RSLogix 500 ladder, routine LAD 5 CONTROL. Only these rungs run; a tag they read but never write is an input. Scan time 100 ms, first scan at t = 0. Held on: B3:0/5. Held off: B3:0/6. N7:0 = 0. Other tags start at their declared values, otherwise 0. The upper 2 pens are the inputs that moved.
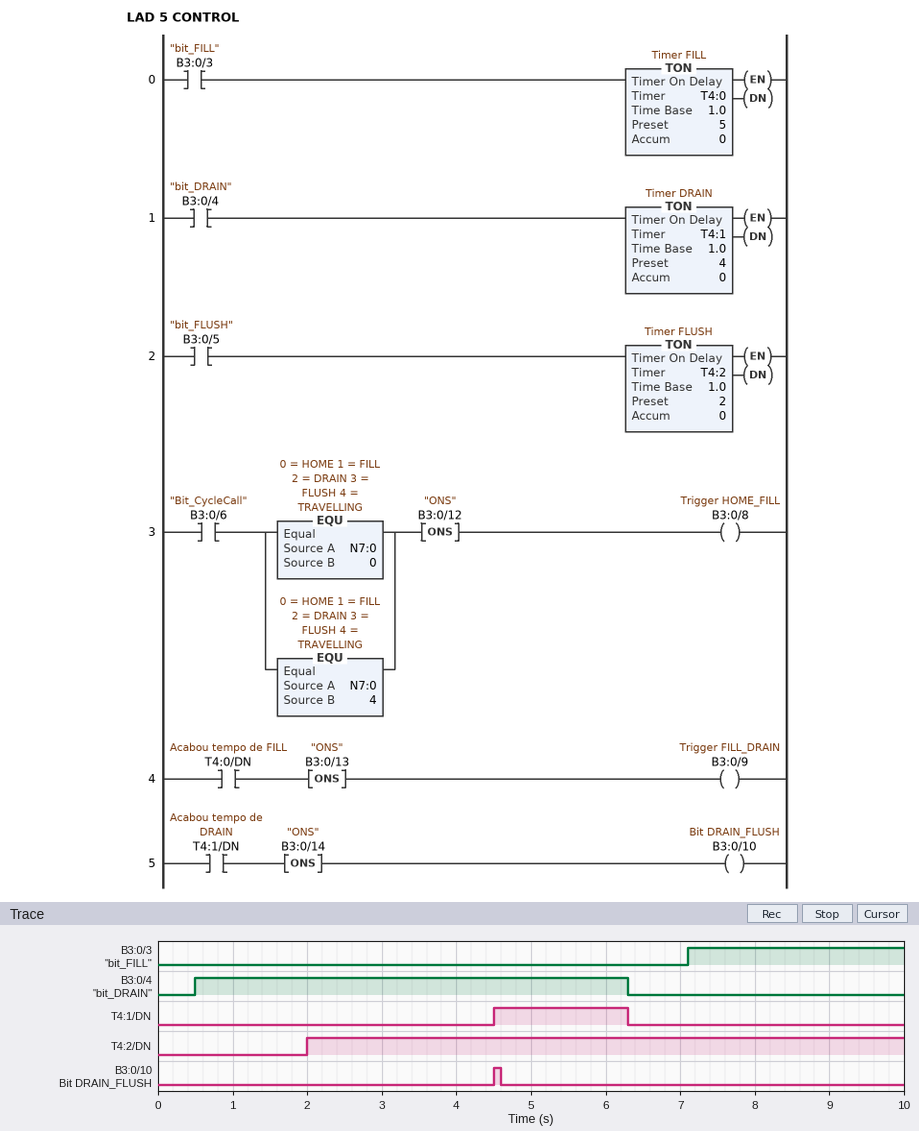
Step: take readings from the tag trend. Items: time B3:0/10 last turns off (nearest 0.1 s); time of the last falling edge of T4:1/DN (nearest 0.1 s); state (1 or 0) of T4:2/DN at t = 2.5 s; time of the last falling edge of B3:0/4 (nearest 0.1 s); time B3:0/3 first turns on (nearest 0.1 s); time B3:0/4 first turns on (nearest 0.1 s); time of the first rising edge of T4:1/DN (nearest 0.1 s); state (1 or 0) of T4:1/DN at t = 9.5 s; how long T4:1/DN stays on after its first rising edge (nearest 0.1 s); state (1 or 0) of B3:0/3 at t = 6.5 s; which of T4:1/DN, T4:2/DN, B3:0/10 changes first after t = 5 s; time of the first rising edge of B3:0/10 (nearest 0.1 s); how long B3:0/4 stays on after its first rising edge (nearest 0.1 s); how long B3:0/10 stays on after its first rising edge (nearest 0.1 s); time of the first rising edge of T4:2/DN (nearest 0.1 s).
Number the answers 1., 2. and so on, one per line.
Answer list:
1. 4.6 s
2. 6.3 s
3. 1
4. 6.3 s
5. 7.1 s
6. 0.5 s
7. 4.5 s
8. 0
9. 1.8 s
10. 0
11. T4:1/DN
12. 4.5 s
13. 5.8 s
14. 0.1 s
15. 2.0 s
